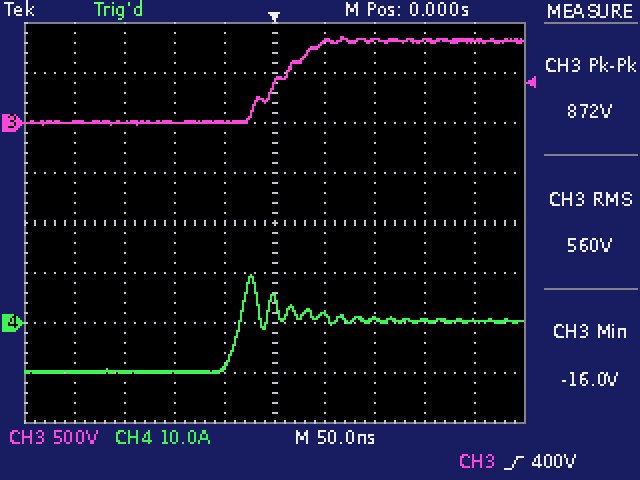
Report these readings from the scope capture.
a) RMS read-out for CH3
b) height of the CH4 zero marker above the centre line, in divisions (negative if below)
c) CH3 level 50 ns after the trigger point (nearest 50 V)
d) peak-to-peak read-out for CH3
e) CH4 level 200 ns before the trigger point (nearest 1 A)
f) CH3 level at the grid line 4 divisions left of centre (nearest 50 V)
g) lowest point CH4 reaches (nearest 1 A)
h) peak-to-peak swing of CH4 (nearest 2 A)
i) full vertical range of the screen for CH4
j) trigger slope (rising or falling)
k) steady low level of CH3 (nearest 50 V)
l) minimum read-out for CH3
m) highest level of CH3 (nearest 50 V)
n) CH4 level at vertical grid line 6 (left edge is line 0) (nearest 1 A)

560 V
-2.0 div
800 V
872 V
-10 A
0 V
-10 A
20 A
80 A
rising
0 V
-16.0 V
850 V
2 A
